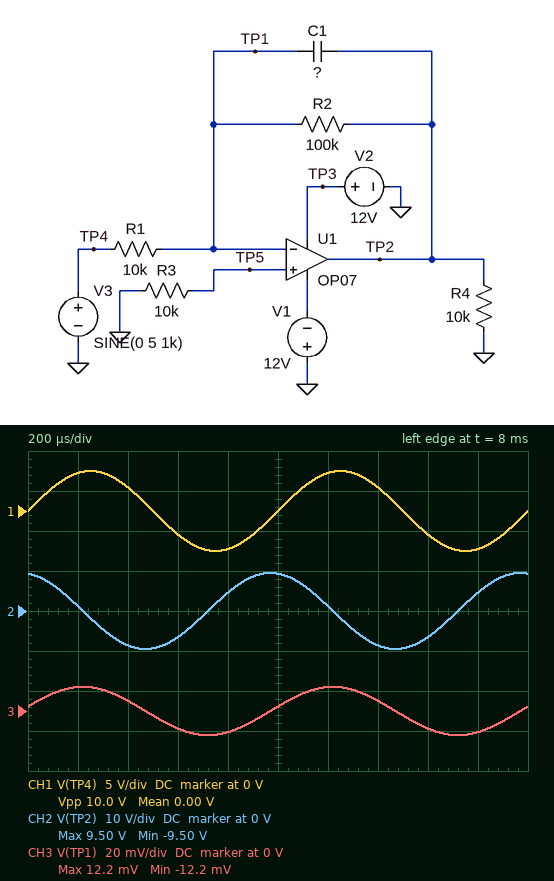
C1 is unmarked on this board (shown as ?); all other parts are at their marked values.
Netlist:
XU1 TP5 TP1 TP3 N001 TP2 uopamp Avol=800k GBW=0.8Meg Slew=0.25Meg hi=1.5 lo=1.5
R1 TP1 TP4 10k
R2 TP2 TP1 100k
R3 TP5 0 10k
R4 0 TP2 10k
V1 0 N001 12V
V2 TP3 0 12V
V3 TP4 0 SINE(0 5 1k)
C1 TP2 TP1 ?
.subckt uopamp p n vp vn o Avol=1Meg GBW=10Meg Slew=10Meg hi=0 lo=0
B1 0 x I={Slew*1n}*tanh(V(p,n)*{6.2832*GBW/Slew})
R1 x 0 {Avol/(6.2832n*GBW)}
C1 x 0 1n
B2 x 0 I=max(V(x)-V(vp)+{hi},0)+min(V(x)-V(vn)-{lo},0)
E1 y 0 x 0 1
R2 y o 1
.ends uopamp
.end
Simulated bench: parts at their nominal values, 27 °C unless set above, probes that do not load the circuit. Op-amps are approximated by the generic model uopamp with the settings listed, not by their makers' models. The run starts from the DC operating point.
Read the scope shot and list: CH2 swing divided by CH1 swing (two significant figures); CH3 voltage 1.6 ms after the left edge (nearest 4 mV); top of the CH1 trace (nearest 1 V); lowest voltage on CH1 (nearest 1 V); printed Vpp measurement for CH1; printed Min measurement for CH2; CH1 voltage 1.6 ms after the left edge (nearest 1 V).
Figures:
1.9
-8 mV
5 V
-5 V
10.0 V
-9.50 V
-3 V
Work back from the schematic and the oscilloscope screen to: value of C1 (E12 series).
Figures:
8.2 nF
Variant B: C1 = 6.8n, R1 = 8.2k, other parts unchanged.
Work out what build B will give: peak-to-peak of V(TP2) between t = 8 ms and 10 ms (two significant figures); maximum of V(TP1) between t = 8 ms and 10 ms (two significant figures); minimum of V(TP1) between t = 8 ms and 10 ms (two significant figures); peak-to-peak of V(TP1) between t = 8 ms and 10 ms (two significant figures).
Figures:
21 V
1.9 V
-1.9 V
3.9 V
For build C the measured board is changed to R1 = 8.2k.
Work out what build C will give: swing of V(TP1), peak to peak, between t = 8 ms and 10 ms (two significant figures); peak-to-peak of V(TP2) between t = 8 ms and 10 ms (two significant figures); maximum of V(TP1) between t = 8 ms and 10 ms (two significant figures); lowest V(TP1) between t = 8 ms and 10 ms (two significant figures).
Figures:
1.7 V
21 V
840 mV
-840 mV
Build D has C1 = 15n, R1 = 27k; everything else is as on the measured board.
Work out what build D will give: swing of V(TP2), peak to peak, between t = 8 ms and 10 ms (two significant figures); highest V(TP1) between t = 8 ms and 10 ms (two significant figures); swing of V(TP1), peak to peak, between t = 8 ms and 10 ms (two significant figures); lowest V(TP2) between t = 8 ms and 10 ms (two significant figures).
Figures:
3.9 V
2.4 mV
4.9 mV
-2.0 V
